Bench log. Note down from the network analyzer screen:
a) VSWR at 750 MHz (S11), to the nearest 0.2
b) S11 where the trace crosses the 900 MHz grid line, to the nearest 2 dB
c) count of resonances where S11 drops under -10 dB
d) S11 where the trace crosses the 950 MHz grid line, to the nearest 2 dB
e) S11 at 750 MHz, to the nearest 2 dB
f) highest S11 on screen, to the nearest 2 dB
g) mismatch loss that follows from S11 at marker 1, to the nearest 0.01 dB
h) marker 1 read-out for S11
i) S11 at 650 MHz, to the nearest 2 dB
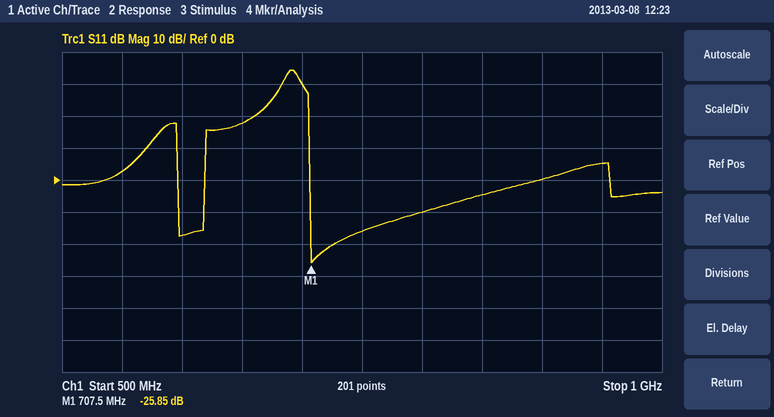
1.4
0 dB
2
6 dB
-16 dB
34 dB
0.01 dB
-25.85 dB
18 dB
